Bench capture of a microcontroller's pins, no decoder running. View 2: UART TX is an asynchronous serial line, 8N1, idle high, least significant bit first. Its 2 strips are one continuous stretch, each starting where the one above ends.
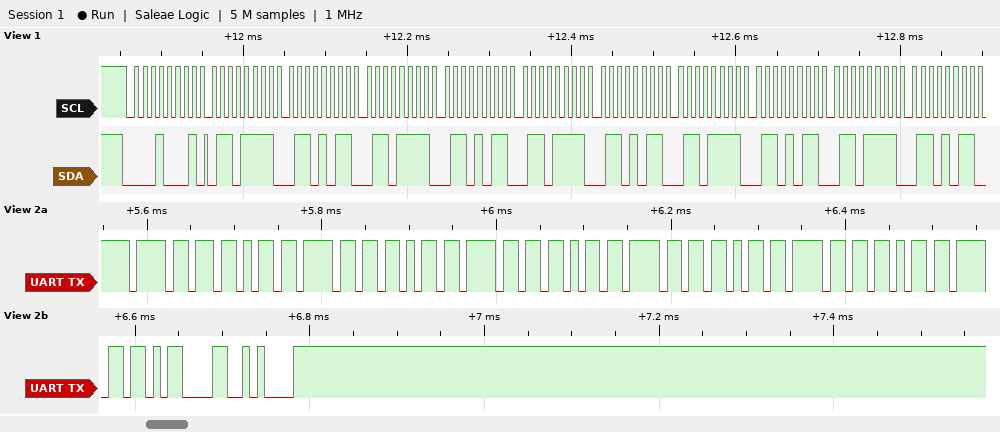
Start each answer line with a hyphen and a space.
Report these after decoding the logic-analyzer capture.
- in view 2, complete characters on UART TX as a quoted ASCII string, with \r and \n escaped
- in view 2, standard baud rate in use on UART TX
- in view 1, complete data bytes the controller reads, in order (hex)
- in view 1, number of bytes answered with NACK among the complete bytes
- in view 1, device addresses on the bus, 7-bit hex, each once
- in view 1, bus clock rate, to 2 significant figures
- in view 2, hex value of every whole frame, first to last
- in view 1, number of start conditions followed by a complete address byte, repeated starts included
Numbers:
- "okokokokoko\r\n"
- 115200 baud
- 6F 6B 6F 6B 6F 6B 6F 6B 6F 6B
- 0
- 0x08
- 100 kHz
- 0x6F 0x6B 0x6F 0x6B 0x6F 0x6B 0x6F 0x6B 0x6F 0x6B 0x6F 0x0D 0x0A
- 1
